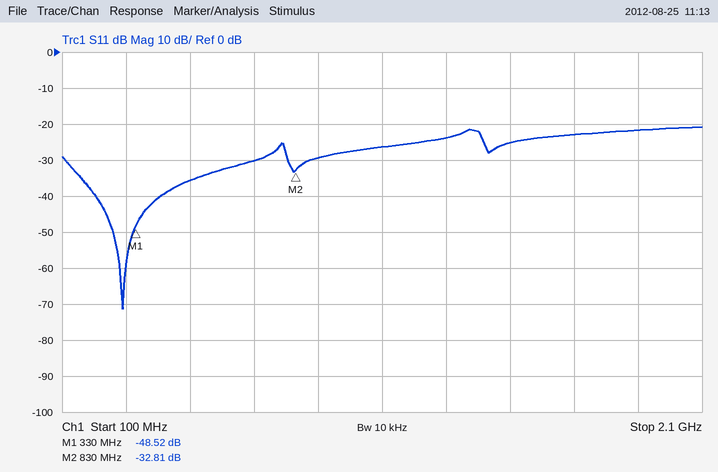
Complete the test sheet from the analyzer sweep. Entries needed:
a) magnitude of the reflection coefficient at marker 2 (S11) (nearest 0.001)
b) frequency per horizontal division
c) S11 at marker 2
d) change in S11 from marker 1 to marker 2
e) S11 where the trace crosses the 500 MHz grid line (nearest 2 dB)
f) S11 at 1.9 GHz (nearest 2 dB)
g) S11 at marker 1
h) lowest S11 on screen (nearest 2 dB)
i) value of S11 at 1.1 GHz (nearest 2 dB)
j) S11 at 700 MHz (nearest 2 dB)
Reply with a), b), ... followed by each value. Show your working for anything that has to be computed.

a) 10^(-32.81/20) ≈ 0.023
b) 200 MHz
c) -32.81 dB
d) -32.81 − (-48.52) = 15.71 dB
e) -36 dB
f) -22 dB
g) -48.52 dB
h) -72 dB
i) -26 dB
j) -30 dB
